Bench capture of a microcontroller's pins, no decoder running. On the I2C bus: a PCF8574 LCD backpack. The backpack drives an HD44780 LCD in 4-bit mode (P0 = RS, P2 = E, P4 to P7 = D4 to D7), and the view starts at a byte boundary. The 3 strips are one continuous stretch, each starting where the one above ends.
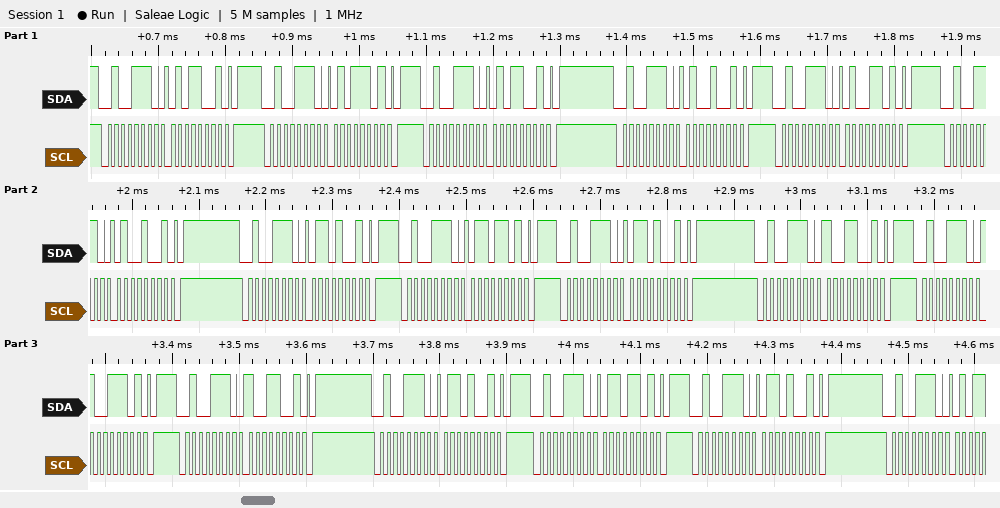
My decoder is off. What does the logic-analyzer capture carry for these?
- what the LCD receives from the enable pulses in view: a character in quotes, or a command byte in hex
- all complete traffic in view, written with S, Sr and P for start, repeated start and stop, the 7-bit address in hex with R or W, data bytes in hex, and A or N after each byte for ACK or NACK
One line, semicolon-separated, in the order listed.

'T' 'i'; S 27W A 59 A P S 27W A 5D A P S 27W A 59 A P S 27W A 49 A P S 27W A 4D A P S 27W A 49 A P S 27W A 69 A P S 27W A 6D A P S 27W A 69 A P S 27W A 99 A P S 27W A 9D A P S 27W A 99 A P S 27W A 69 A P S 27W A 6D A P S 27W A 69 A P S 27W A
